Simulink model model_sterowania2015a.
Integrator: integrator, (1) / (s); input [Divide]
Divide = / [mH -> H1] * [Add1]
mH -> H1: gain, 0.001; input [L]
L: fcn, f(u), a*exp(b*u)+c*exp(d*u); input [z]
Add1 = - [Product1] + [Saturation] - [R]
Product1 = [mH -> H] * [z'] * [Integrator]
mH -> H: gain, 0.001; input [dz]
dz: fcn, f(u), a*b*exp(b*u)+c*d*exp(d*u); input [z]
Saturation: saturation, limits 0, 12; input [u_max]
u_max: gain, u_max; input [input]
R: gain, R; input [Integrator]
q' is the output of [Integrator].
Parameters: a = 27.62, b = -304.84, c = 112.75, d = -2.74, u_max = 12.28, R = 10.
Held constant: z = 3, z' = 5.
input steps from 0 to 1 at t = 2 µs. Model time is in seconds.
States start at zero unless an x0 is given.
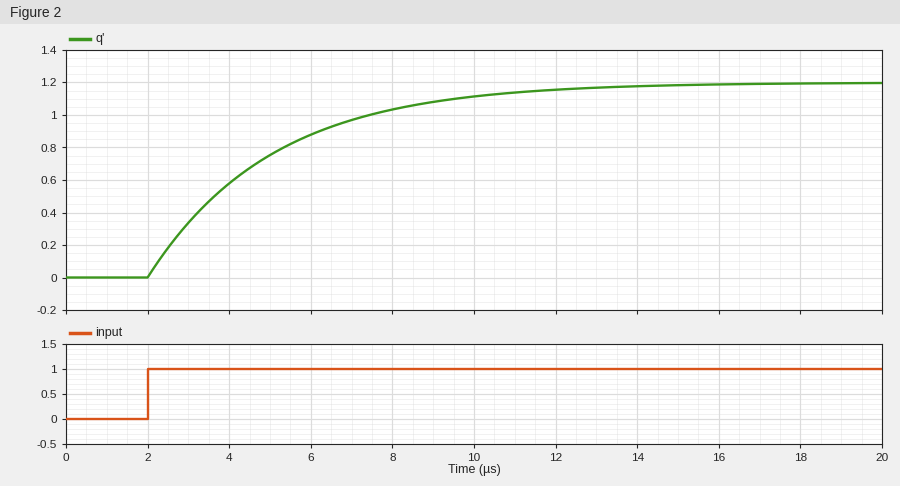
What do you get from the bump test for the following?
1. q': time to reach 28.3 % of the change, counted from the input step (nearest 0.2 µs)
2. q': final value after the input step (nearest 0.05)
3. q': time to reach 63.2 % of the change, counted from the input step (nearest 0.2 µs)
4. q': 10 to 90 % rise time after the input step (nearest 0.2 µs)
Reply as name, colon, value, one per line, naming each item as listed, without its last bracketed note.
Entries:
q': time to reach 28.3 % of the change, counted from the input step: 1.0 µs
q': final value after the input step: 1.20
q': time to reach 63.2 % of the change, counted from the input step: 3.0 µs
q': 10 to 90 % rise time after the input step: 6.6 µs
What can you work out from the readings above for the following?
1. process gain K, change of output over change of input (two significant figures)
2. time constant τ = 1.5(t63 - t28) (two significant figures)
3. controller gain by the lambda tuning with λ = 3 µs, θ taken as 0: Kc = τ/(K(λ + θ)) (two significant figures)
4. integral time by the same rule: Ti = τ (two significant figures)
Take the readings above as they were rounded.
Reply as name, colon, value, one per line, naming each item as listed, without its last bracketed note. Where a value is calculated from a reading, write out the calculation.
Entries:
process gain K, change of output over change of input: (1.2 - 0) / 1 = 1.2
time constant τ = 1.5(t63 - t28): 1.5 × (3 - 1) = 3.0 µs
controller gain by the lambda tuning with λ = 3 µs, θ taken as 0: Kc = τ/(K(λ + θ)): 3 / (1.2 × (3 + 0)) = 0.83
integral time by the same rule: Ti = τ: 3.0 µs
